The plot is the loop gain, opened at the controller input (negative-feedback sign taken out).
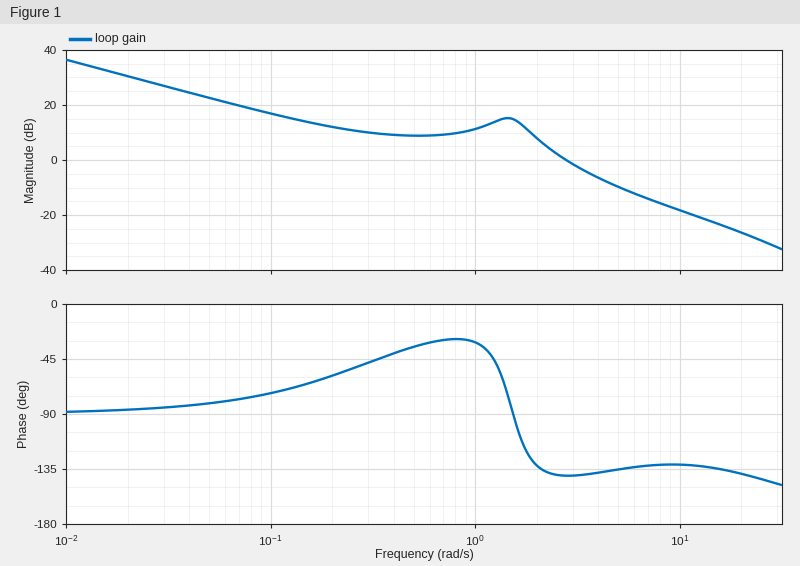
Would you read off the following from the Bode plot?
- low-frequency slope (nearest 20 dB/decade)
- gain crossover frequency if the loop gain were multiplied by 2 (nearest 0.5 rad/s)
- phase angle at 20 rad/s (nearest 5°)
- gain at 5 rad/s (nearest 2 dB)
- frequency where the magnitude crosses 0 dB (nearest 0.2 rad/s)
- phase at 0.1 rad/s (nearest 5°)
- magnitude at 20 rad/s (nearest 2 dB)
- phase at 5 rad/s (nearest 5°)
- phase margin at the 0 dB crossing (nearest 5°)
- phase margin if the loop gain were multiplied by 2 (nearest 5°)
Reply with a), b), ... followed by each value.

a) -20 dB/decade
b) 4.0 rad/s
c) -140°
d) -10 dB
e) 2.8 rad/s
f) -75°
g) -26 dB
h) -135°
i) 40°
j) 40°
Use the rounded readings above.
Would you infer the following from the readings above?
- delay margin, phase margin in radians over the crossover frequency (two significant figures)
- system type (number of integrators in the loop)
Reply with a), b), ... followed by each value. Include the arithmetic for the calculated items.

a) 40 × π / 180 / 2.8 = 0.25 s
b) 1
